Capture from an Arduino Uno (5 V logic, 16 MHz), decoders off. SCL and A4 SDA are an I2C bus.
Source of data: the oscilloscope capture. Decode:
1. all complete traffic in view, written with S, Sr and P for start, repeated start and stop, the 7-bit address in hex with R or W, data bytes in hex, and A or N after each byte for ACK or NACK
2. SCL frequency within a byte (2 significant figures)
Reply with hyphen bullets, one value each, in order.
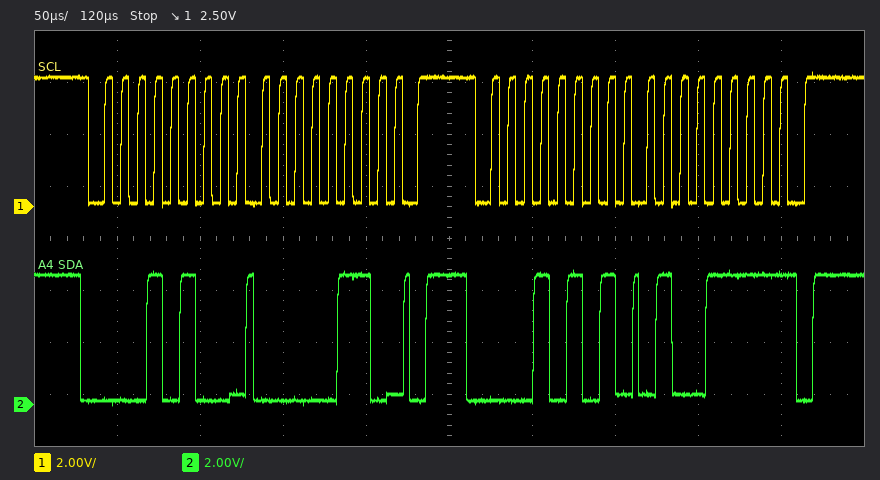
- S 0AW A 06 A P S 0AR A 4F N P
- 100 kHz
